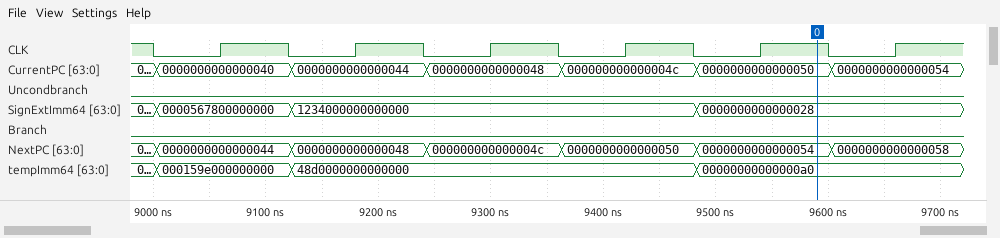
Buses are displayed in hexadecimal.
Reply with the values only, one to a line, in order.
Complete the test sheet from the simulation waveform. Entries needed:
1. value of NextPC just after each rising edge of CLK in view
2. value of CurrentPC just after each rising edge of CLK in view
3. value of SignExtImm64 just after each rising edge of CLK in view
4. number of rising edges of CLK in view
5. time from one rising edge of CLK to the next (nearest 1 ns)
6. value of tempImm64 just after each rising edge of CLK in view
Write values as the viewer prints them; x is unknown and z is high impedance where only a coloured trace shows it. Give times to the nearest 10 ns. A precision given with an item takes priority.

0000000000000044, 0000000000000048, 000000000000004c, 0000000000000050, 0000000000000054, 0000000000000058
0000000000000040, 0000000000000044, 0000000000000048, 000000000000004c, 0000000000000050, 0000000000000054
0000567800000000, 1234000000000000, 1234000000000000, 1234000000000000, 0000000000000028, 0000000000000028
6
120 ns
000159e000000000, 48d0000000000000, 48d0000000000000, 48d0000000000000, 00000000000000a0, 00000000000000a0
